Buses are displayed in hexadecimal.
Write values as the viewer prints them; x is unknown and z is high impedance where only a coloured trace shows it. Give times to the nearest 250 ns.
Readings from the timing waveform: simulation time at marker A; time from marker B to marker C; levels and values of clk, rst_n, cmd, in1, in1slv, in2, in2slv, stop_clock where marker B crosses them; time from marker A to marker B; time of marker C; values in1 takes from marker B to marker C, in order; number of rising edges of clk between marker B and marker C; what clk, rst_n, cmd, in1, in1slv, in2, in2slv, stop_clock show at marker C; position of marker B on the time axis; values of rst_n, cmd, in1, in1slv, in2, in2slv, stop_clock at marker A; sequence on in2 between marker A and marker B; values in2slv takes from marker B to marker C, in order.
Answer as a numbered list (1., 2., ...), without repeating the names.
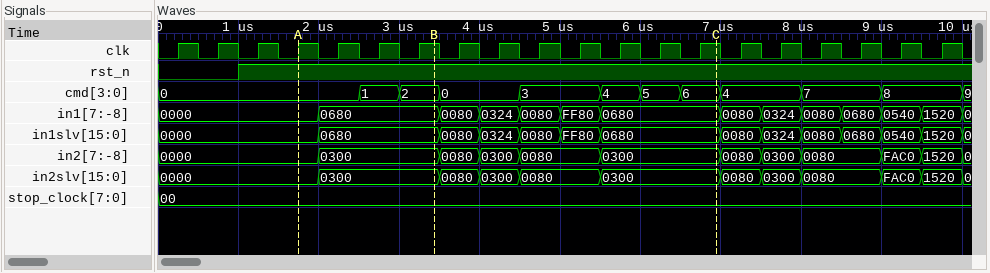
1. 1750 ns
2. 3500 ns
3. clk=1, rst_n=1, cmd=2, in1=0680, in1slv=0680, in2=0300, in2slv=0300, stop_clock=00
4. 1750 ns
5. 7000 ns
6. 0680, 0080, 0324, 0080, FF80, 0680
7. 7
8. clk=1, rst_n=1, cmd=6, in1=0680, in1slv=0680, in2=0300, in2slv=0300, stop_clock=00
9. 3500 ns
10. rst_n=1, cmd=0, in1=0000, in1slv=0000, in2=0000, in2slv=0000, stop_clock=00
11. 0000, 0300
12. 0300, 0080, 0300, 0080, 0300
